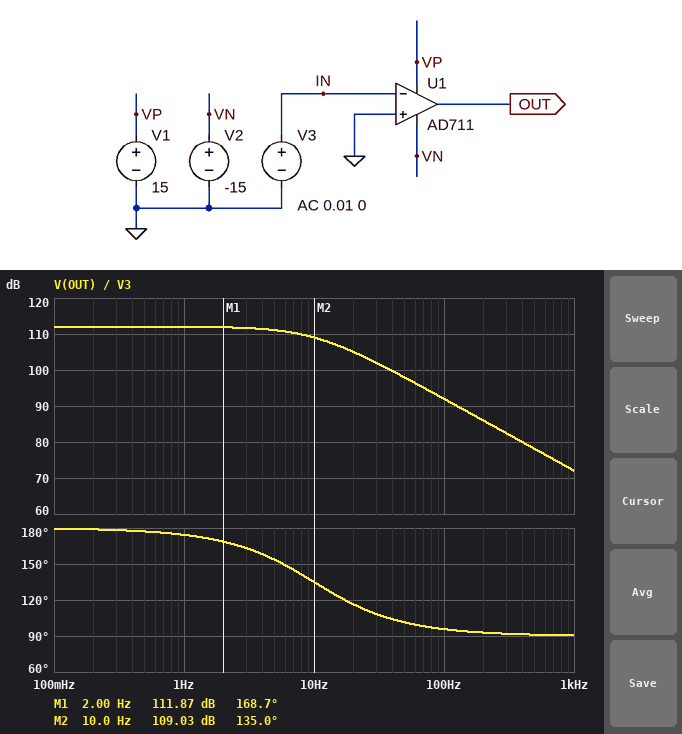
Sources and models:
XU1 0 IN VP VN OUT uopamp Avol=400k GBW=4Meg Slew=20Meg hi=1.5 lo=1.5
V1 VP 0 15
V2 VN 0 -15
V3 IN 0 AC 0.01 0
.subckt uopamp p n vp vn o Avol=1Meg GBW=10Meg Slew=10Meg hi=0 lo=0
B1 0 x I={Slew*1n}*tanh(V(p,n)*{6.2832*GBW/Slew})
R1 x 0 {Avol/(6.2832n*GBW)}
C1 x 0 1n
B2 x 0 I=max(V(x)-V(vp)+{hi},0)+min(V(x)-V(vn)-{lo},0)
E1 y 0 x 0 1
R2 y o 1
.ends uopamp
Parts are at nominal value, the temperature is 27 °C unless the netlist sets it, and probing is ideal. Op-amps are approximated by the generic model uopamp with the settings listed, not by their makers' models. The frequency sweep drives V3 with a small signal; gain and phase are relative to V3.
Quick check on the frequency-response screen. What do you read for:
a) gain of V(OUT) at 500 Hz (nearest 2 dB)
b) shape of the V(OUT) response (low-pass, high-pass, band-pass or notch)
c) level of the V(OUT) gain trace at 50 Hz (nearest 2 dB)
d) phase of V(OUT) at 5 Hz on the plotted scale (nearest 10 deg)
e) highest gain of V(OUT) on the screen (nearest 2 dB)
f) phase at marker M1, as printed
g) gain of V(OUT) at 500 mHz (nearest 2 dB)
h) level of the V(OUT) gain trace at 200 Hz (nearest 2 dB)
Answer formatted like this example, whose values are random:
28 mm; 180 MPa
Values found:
78 dB; low-pass; 98 dB; 150 deg; 112 dB; 168.7 deg; 112 dB; 86 dB
